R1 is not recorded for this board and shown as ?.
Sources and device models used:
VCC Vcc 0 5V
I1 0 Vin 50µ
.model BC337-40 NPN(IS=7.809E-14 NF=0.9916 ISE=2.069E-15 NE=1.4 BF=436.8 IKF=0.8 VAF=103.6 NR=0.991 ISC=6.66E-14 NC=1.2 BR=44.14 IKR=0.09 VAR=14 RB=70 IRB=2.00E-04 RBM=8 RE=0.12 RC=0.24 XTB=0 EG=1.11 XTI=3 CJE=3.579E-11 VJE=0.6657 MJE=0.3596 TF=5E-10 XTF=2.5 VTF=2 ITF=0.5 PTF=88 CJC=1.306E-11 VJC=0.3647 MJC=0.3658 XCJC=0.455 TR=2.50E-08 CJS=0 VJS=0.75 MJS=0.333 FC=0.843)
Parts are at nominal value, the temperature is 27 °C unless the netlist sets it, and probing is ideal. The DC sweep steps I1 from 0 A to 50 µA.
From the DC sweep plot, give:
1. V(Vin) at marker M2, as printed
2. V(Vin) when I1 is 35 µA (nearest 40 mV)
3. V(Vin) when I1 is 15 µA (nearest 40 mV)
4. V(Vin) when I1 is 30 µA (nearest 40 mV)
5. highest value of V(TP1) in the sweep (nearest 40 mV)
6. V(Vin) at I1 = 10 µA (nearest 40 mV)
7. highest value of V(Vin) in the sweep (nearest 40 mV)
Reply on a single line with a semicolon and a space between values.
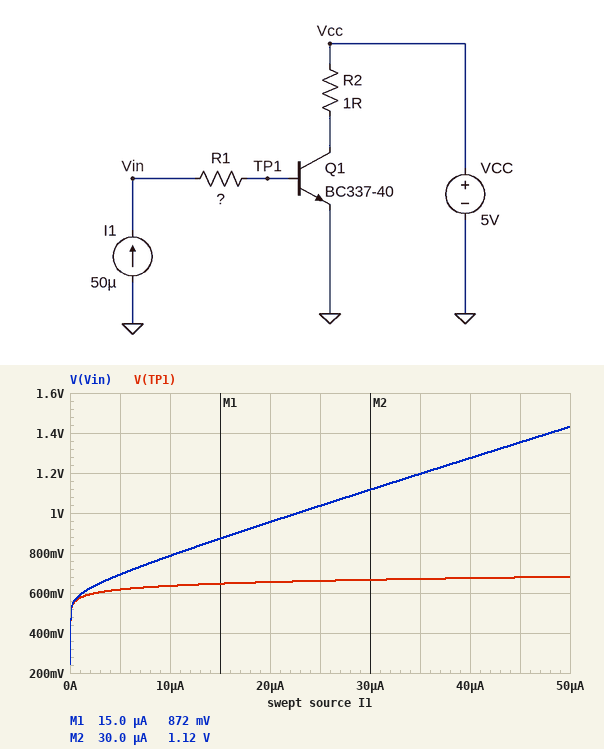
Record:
1.12 V; 1.20 V; 880 mV; 1.12 V; 680 mV; 800 mV; 1.44 V
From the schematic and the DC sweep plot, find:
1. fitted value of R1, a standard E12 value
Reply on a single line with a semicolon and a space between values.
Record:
15 kΩ
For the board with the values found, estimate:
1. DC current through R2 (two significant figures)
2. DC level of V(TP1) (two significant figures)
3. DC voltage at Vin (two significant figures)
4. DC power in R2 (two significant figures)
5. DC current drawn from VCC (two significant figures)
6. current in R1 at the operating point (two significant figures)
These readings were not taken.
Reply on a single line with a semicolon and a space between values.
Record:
21 mA; 680 mV; 1.4 V; 440 µW; 21 mA; 50 µA
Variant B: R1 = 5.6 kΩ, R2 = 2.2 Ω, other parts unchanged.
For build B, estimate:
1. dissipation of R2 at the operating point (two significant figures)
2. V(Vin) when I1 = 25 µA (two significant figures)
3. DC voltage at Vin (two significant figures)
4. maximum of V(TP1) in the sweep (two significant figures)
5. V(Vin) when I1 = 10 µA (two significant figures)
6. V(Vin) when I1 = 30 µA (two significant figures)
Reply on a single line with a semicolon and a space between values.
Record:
970 µW; 800 mV; 960 mV; 680 mV; 690 mV; 830 mV
